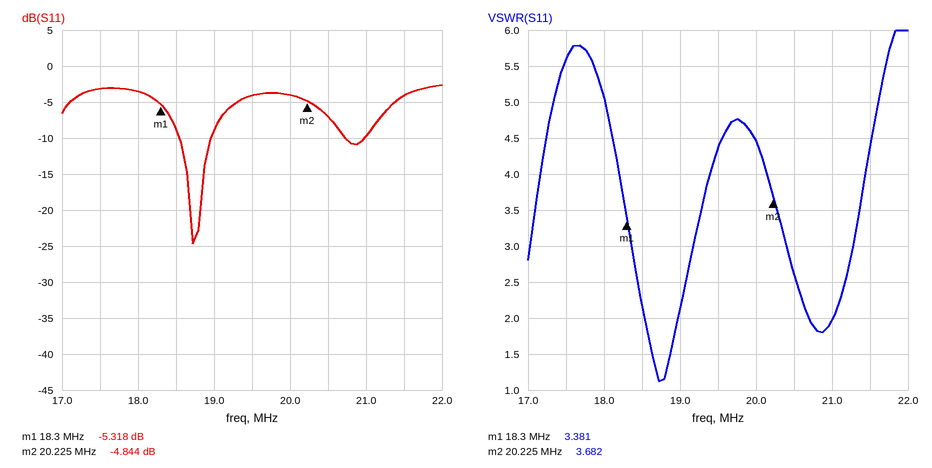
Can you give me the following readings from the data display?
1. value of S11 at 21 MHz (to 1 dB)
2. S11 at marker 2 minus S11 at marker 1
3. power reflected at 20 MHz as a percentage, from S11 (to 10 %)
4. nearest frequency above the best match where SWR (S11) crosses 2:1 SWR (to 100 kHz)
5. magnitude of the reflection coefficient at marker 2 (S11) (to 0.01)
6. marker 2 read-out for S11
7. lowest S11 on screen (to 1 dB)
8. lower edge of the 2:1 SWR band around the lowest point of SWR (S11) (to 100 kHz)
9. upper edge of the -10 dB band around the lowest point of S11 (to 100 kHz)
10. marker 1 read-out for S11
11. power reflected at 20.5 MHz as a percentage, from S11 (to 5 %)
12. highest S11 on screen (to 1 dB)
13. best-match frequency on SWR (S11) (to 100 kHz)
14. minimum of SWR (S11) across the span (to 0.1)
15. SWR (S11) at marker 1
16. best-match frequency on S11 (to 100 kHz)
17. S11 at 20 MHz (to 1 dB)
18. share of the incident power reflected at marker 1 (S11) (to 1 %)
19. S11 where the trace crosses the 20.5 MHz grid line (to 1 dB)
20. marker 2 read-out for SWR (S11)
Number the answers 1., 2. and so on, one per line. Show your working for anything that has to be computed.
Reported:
1. -10 dB
2. -4.844 − (-5.318) = 0.474 dB
3. 10^(-4/10) ≈ 40 %
4. 19.0 MHz
5. 10^(-4.844/20) ≈ 0.57
6. -4.844 dB
7. -25 dB
8. 18.5 MHz
9. 19.0 MHz
10. -5.318 dB
11. 10^(-7/10) ≈ 20 %
12. -3 dB
13. 18.7 MHz
14. 1.1
15. 3.381
16. 18.7 MHz
17. -4 dB
18. 10^(-5.318/10) ≈ 29 %
19. -7 dB
20. 3.682
